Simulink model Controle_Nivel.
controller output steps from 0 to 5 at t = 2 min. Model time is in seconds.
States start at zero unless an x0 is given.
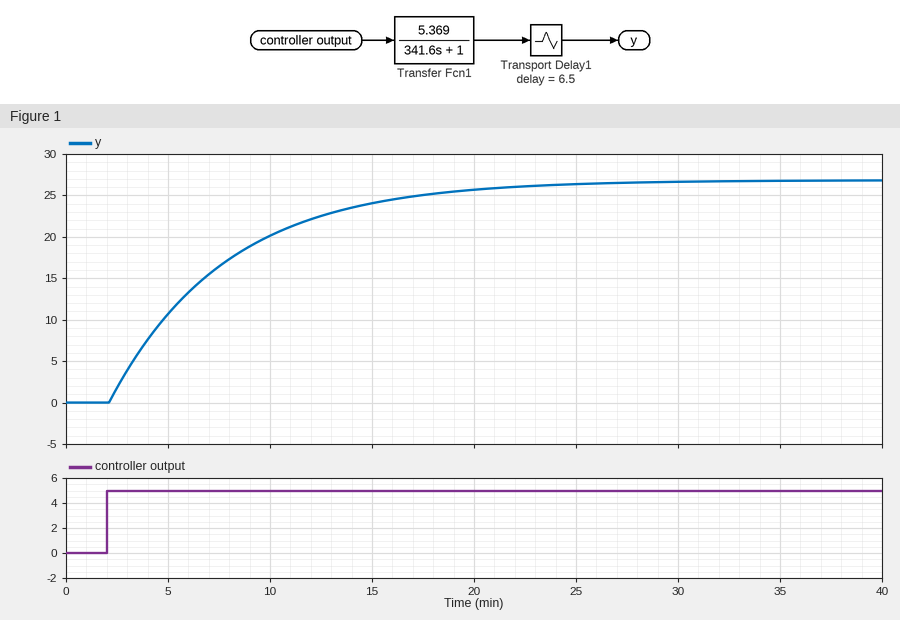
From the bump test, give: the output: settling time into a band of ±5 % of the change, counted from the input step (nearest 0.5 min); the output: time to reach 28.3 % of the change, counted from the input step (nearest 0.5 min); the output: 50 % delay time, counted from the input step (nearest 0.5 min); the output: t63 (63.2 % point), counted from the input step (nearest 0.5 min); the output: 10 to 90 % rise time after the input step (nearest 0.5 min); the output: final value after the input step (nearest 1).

17.0 min
2.0 min
4.0 min
6.0 min
12.5 min
27
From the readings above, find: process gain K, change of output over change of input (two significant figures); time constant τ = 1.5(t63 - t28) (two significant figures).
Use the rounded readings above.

5.4
6.0 min
